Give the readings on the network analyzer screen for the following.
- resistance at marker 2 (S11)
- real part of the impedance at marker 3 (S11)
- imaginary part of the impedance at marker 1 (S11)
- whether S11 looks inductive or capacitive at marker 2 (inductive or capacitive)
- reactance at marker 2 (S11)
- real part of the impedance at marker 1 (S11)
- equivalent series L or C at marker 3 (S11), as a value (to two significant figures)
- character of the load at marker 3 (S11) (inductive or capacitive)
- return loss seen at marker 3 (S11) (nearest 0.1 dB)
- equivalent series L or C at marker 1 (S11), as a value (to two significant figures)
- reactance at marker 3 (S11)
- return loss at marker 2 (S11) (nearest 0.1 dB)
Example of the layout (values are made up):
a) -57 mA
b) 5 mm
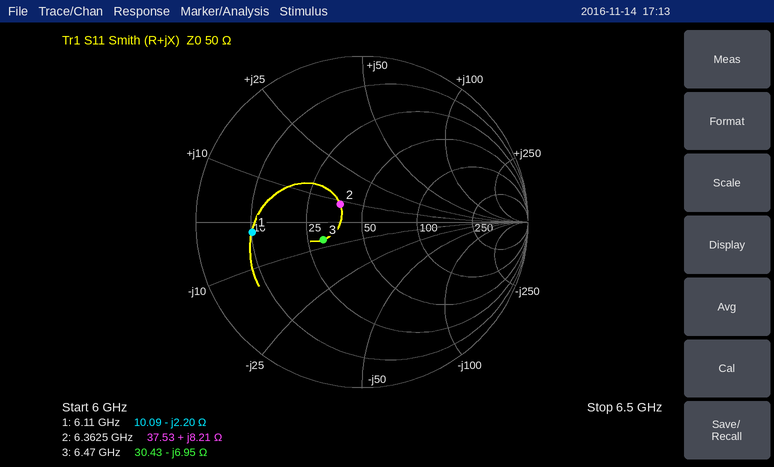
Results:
a) 37.53 Ω
b) 30.43 Ω
c) -2.20 Ω
d) inductive
e) +8.21 Ω
f) 10.09 Ω
g) 3.5 pF
h) capacitive
i) 11.8 dB
j) 12 pF
k) -6.95 Ω
l) 15.4 dB
